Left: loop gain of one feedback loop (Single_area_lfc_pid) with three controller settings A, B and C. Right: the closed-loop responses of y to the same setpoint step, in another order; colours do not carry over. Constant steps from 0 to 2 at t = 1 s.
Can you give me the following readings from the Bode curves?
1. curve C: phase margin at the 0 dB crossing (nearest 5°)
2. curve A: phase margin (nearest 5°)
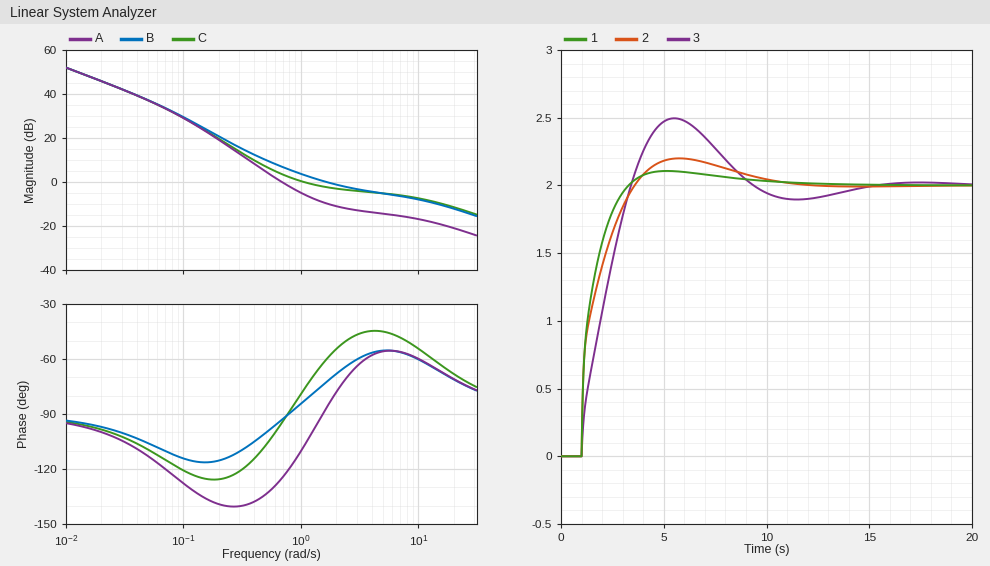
105°
55°
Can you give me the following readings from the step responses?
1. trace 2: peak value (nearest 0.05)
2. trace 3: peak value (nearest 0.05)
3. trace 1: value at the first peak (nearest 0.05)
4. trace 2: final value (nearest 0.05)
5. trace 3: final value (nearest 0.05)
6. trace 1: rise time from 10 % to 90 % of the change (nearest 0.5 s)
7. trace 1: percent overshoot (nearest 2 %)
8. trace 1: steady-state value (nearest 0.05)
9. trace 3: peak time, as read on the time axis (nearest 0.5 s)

2.20
2.50
2.10
2.00
2.00
1.5 s
6 %
2.00
5.5 s
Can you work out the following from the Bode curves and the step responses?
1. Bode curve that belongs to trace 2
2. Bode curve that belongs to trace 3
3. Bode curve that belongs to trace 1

C
A
B
